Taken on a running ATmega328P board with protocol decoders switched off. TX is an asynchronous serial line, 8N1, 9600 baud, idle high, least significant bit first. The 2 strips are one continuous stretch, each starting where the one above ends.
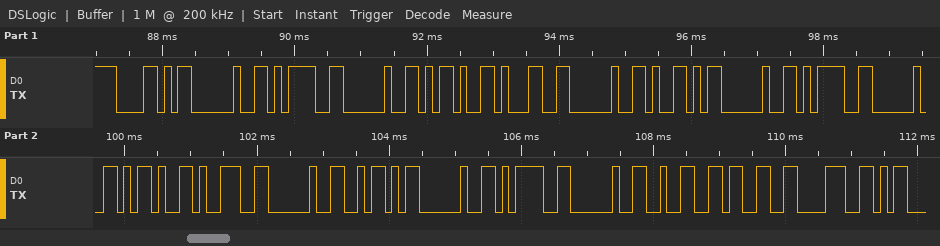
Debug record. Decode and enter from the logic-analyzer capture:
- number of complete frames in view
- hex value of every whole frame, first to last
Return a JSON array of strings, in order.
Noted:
["21", "0x58 0x20 0x3D 0x20 0x2D 0x31 0x20 0x59 0x20 0x3D 0x20 0x2D 0x39 0x20 0x5A 0x20 0x3D 0x20 0x32 0x33 0x38"]
